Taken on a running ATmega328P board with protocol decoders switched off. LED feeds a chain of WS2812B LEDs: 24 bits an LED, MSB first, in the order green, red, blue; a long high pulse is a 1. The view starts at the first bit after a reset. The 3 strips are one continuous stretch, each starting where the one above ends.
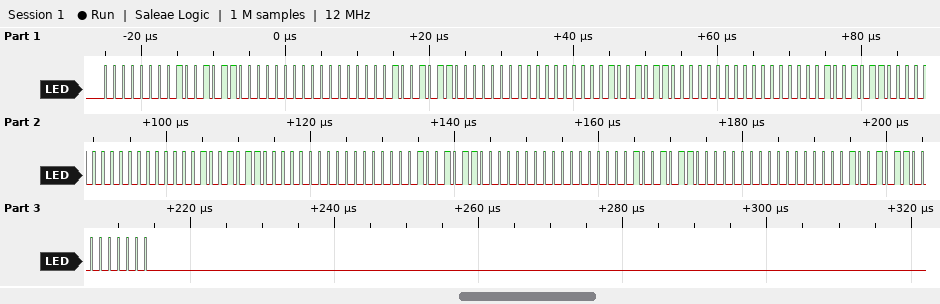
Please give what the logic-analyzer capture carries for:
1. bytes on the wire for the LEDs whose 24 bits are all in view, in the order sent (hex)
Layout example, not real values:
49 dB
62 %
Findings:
00 96 00 00 96 00 00 96 00 00 96 00 00 96 00 00 96 00 00 96 00 00 96 00
